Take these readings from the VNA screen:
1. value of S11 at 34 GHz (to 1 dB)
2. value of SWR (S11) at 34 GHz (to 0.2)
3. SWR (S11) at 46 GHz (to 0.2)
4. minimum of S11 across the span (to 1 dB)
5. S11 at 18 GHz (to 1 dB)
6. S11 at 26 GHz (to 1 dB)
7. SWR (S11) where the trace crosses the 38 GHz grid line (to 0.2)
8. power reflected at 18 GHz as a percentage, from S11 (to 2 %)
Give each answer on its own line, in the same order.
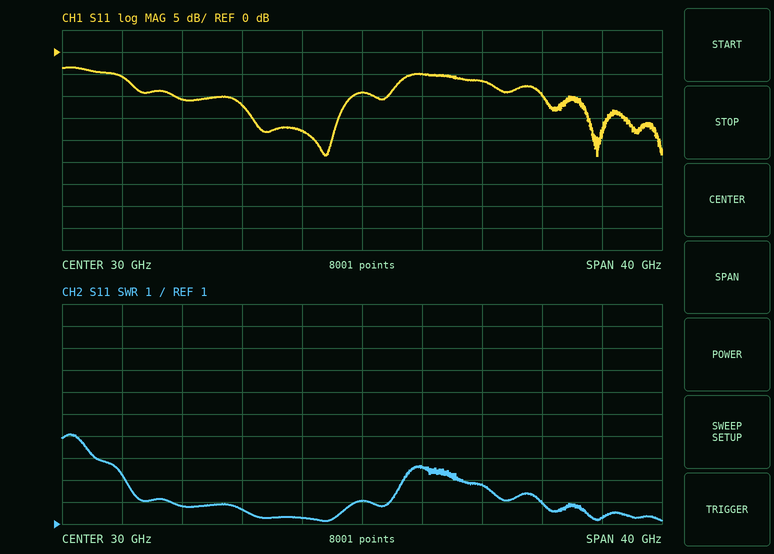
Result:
-5 dB
3.6
1.2
-24 dB
-11 dB
-18 dB
2.8
8 %
